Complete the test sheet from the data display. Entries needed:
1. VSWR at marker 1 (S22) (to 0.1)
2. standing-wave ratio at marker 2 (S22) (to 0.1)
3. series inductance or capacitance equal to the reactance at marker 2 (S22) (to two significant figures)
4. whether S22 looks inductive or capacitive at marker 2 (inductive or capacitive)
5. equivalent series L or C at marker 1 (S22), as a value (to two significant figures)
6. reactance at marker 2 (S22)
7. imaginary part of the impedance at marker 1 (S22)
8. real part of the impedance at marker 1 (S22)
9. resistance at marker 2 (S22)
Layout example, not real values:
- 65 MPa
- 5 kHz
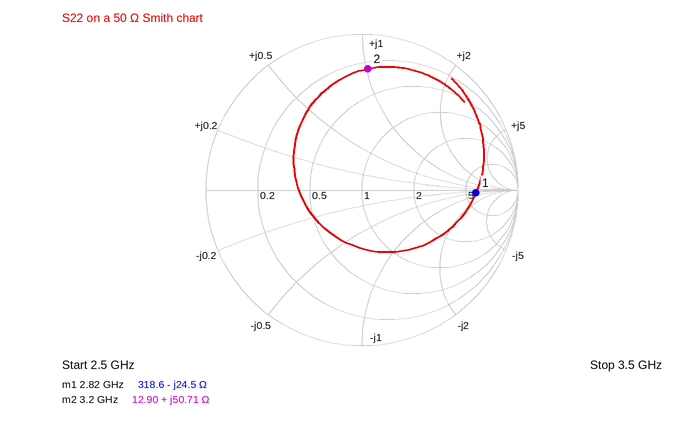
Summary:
- 6.4
- 8.0
- 2.5 nH
- inductive
- 2.3 pF
- +50.71 Ω
- -24.5 Ω
- 318.6 Ω
- 12.90 Ω
